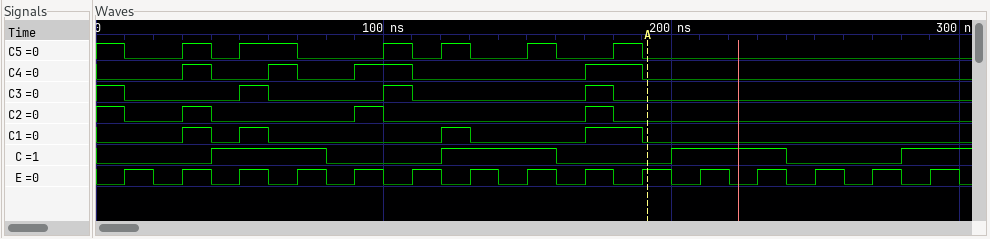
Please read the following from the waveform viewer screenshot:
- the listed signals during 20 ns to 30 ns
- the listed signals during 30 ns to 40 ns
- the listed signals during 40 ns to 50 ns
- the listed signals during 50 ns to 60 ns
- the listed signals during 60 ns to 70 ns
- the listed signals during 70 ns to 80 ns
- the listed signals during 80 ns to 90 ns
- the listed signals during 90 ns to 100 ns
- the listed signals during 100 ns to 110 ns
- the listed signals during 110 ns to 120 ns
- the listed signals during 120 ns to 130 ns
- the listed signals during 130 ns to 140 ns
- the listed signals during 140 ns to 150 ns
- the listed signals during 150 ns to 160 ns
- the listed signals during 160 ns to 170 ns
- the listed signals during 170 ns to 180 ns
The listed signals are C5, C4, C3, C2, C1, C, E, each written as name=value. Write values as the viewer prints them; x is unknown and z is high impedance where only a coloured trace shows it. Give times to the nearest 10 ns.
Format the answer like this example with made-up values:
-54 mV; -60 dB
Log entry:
C5=0, C4=0, C3=0, C2=0, C1=0, C=0, E=0; C5=1, C4=1, C3=0, C2=1, C1=1, C=0, E=1; C5=0, C4=0, C3=0, C2=0, C1=0, C=1, E=0; C5=1, C4=0, C3=1, C2=0, C1=1, C=1, E=1; C5=1, C4=1, C3=0, C2=0, C1=0, C=1, E=0; C5=0, C4=0, C3=0, C2=0, C1=0, C=1, E=1; C5=0, C4=0, C3=0, C2=0, C1=0, C=0, E=0; C5=0, C4=1, C3=0, C2=1, C1=0, C=0, E=1; C5=1, C4=1, C3=1, C2=0, C1=0, C=0, E=0; C5=0, C4=0, C3=0, C2=0, C1=0, C=0, E=1; C5=1, C4=0, C3=0, C2=0, C1=1, C=1, E=0; C5=0, C4=0, C3=0, C2=0, C1=0, C=1, E=1; C5=0, C4=0, C3=0, C2=0, C1=0, C=1, E=0; C5=1, C4=0, C3=0, C2=0, C1=0, C=1, E=1; C5=0, C4=0, C3=0, C2=0, C1=0, C=0, E=0; C5=0, C4=1, C3=1, C2=1, C1=1, C=0, E=1
